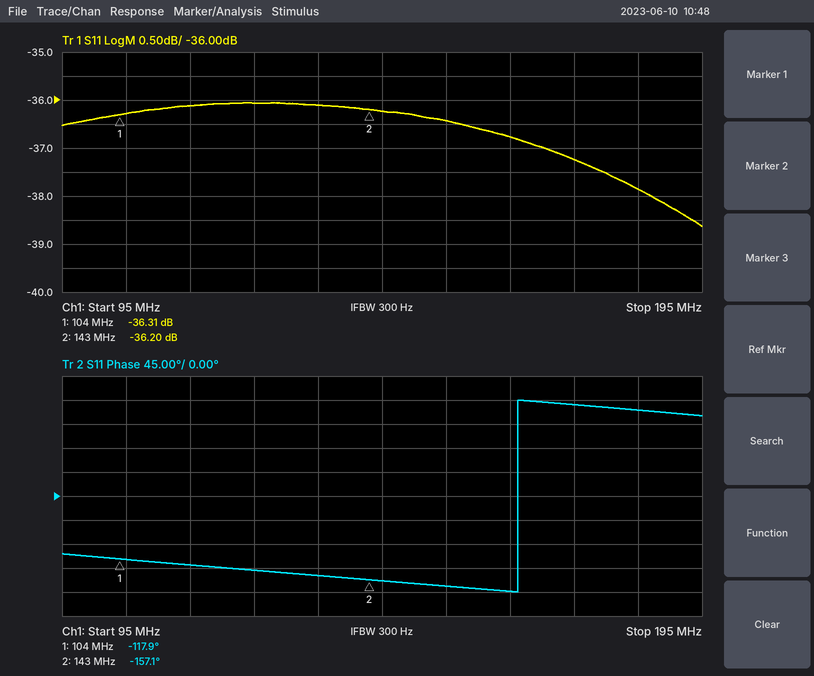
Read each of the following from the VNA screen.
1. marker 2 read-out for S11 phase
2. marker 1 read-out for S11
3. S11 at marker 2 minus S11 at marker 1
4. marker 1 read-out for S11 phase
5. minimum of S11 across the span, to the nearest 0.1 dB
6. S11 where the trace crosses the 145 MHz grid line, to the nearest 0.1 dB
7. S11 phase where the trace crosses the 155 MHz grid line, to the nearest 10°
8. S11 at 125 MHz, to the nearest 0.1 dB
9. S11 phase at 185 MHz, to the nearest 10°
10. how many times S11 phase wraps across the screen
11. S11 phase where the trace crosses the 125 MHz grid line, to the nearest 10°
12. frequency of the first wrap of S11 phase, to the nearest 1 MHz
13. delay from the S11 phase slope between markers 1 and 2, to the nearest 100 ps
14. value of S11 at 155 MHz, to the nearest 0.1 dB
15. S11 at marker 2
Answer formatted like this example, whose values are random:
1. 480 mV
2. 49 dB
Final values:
1. -157.1°
2. -36.31 dB
3. 0.11 dB
4. -117.9°
5. -38.6 dB
6. -36.2 dB
7. -170°
8. -36.1 dB
9. 160°
10. 1
11. -140°
12. 166 MHz
13. 2.8 ns
14. -36.4 dB
15. -36.20 dB
